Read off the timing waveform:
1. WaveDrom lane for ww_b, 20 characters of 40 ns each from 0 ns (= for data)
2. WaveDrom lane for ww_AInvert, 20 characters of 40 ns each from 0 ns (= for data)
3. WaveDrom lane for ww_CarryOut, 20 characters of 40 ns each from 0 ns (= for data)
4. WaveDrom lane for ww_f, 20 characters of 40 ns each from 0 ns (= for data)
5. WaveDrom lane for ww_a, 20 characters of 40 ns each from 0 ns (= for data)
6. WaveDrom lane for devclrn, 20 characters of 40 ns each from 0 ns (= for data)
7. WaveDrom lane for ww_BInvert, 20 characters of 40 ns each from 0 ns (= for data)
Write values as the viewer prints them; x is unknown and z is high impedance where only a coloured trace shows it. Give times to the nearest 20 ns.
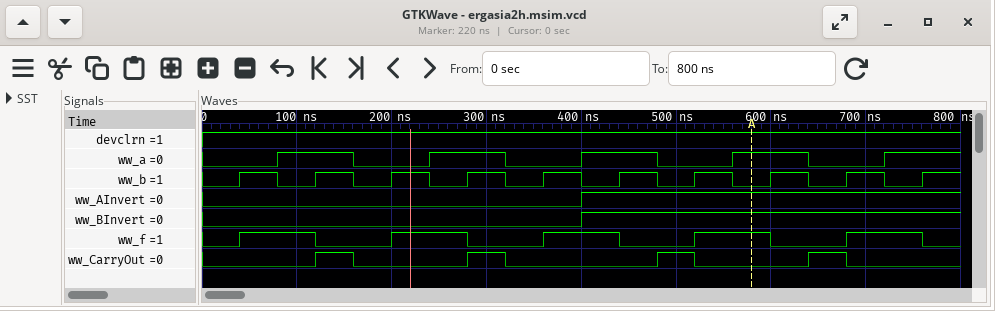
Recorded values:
{name: 'ww_b', wave: '01010101010101010101'}
{name: 'ww_AInvert', wave: '0.........1.........'}
{name: 'ww_CarryOut', wave: '0..10..10...10..10..'}
{name: 'ww_f', wave: '01.0.1.0.1.0.1.0.1.0'}
{name: 'ww_a', wave: '0.1.0.1.0.1.0.1.0.1.'}
{name: 'devclrn', wave: '1...................'}
{name: 'ww_BInvert', wave: '0.........1.........'}
